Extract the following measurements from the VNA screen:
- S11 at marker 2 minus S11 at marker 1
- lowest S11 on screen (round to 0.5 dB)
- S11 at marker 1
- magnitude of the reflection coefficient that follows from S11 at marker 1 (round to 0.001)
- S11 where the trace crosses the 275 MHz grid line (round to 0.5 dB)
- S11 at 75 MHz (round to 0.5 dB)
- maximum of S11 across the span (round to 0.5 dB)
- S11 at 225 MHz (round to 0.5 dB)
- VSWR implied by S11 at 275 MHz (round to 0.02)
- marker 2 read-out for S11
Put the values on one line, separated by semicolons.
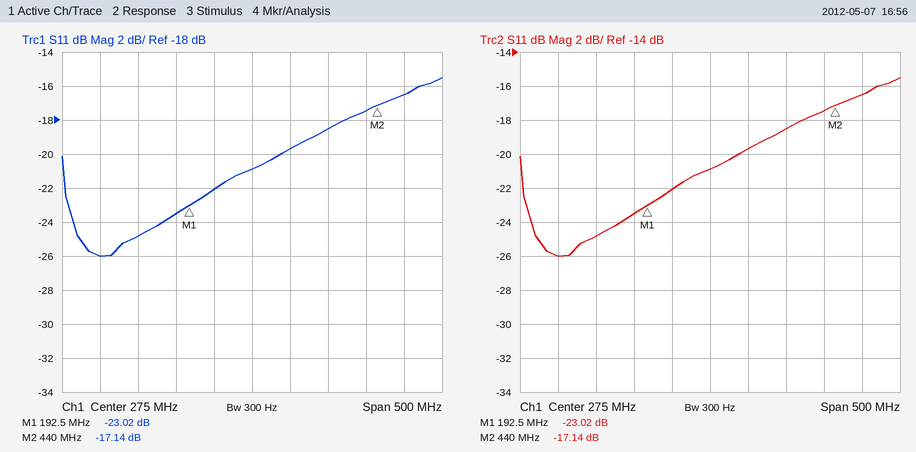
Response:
5.88 dB; -26.0 dB; -23.02 dB; 0.071; -21.0 dB; -26.0 dB; -15.5 dB; -22.0 dB; 1.20; -17.14 dB
